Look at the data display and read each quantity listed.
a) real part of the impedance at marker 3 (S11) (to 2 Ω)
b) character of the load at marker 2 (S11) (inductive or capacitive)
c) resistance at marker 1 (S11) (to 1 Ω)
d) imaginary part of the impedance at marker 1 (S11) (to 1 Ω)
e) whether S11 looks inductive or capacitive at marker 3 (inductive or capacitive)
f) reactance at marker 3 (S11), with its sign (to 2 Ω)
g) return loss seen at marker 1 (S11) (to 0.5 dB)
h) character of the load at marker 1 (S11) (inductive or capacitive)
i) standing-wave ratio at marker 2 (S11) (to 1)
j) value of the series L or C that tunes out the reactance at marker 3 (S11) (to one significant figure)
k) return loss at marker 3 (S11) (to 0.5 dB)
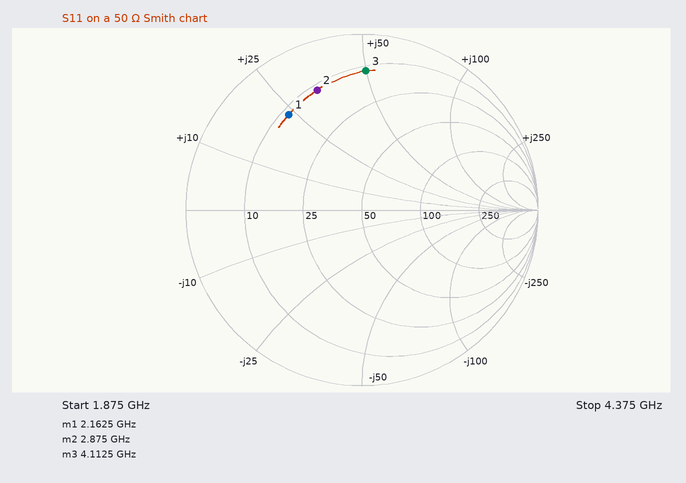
12 Ω
inductive
12 Ω
+24 Ω
inductive
+50 Ω
3.5 dB
inductive
6
800 fF
2.0 dB
